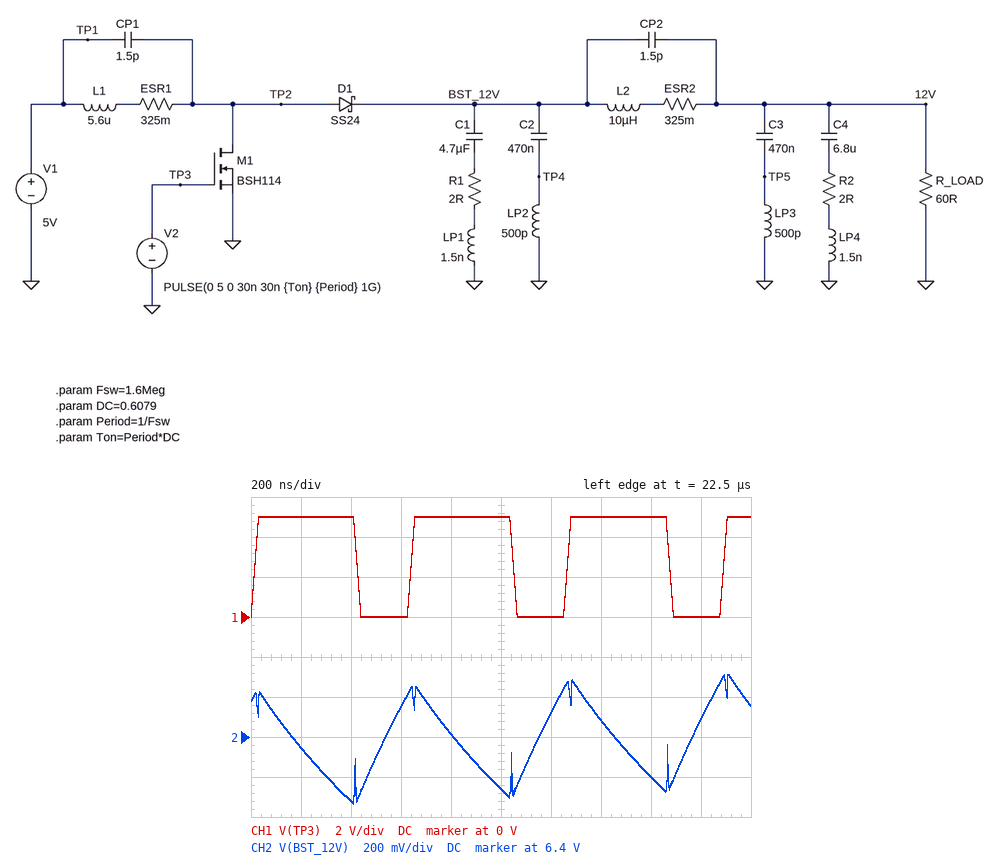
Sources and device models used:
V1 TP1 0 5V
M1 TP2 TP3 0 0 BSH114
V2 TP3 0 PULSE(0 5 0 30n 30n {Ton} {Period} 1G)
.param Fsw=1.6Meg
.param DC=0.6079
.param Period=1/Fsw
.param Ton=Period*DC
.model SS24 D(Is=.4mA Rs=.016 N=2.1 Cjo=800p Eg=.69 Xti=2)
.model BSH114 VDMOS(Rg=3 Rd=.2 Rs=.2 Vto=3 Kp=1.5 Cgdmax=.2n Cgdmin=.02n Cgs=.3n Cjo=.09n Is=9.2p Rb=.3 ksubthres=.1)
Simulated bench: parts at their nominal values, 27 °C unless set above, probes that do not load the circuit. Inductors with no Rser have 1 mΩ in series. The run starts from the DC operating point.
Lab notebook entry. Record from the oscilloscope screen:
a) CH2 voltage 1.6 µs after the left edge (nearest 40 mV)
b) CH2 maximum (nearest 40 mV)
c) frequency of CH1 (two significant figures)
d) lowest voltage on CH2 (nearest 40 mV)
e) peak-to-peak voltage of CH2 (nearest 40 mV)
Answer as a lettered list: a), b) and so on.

a) 6.20 V
b) 6.72 V
c) 1.6 MHz
d) 6.08 V
e) 640 mV
